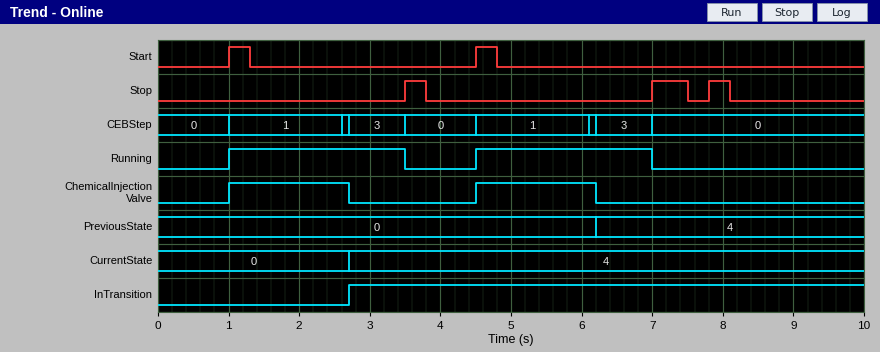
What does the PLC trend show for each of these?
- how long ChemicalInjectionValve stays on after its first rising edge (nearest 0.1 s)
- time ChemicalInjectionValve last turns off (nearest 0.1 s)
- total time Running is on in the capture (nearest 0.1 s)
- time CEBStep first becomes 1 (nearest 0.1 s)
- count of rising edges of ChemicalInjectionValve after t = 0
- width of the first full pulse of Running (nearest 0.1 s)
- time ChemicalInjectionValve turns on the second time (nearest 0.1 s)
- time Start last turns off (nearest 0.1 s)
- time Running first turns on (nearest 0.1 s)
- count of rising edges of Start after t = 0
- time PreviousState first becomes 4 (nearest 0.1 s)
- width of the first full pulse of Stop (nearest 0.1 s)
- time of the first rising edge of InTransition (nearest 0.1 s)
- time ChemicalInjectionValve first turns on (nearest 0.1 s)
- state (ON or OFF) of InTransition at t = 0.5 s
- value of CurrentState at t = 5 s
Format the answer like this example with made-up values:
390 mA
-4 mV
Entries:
1.7 s
6.2 s
5.0 s
1.0 s
2
2.5 s
4.5 s
4.8 s
1.0 s
2
6.2 s
0.3 s
2.7 s
1.0 s
OFF
4
